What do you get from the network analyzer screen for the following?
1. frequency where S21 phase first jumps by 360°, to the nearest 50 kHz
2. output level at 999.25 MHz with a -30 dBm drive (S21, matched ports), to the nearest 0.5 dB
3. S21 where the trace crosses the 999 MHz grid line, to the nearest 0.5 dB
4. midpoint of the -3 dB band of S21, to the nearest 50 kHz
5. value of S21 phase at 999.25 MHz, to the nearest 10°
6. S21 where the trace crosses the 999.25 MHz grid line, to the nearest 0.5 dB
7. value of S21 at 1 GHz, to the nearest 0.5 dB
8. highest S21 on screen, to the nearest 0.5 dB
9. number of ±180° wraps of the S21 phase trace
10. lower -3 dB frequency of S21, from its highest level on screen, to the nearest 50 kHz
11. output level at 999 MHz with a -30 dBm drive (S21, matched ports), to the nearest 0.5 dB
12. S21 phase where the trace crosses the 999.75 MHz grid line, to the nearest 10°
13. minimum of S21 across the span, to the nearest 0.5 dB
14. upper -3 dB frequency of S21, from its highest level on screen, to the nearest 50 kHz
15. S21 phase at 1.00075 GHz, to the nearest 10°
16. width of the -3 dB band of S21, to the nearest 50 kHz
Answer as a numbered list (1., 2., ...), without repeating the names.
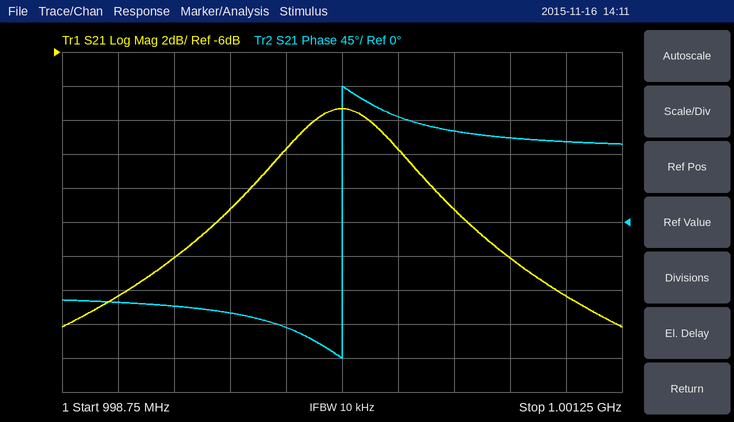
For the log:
1. 1.00000 GHz
2. -48.0 dBm
3. -20.5 dB
4. 1.00000 GHz
5. -110°
6. -18.0 dB
7. -9.5 dB
8. -9.5 dB
9. 1
10. 999.70 MHz
11. -50.5 dBm
12. -140°
13. -22.0 dB
14. 1.00030 GHz
15. 110°
16. 600 kHz
